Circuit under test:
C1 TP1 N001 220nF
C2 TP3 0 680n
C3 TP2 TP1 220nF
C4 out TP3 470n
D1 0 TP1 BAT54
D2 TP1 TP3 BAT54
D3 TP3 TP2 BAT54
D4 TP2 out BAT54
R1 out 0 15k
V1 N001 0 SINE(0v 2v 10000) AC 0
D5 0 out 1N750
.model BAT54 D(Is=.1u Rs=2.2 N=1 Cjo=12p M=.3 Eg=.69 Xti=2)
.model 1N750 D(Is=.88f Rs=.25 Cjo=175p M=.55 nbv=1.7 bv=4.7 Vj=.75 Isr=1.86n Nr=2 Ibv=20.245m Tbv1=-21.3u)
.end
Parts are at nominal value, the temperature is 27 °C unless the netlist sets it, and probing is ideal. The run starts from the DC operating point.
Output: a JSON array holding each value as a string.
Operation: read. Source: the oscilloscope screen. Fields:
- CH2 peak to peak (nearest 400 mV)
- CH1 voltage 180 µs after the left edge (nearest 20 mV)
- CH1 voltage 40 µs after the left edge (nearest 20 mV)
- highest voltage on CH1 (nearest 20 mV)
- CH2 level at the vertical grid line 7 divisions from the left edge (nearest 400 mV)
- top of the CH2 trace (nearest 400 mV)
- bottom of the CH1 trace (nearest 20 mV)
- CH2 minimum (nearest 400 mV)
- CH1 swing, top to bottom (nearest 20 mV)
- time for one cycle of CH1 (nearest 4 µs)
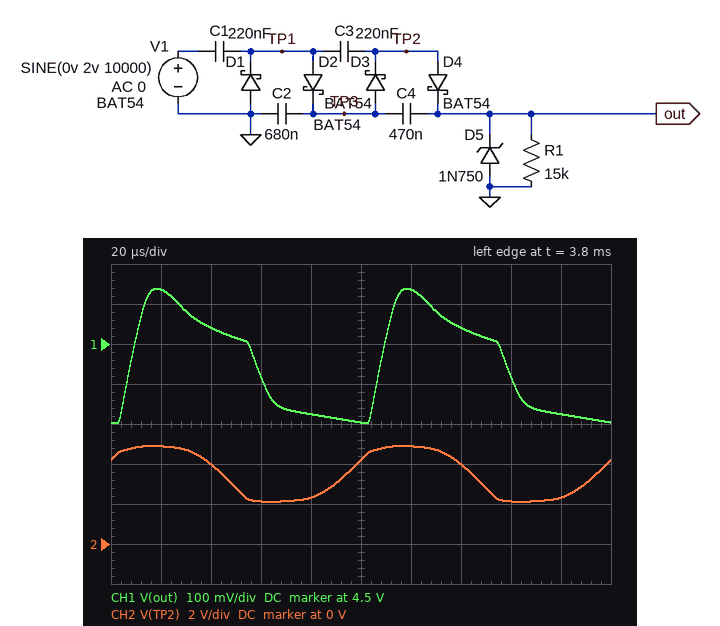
["2.8 V", "4.32 V", "4.54 V", "4.64 V", "4.0 V", "4.8 V", "4.30 V", "2.0 V", "340 mV", "100 µs"]
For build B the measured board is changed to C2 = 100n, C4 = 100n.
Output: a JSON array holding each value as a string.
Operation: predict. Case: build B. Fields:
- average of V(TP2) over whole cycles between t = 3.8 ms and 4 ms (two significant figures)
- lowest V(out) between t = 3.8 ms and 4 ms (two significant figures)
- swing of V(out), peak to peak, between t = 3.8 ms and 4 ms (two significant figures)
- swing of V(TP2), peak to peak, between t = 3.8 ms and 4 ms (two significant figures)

["3.3 V", "3.4 V", "1.2 V", "3.2 V"]
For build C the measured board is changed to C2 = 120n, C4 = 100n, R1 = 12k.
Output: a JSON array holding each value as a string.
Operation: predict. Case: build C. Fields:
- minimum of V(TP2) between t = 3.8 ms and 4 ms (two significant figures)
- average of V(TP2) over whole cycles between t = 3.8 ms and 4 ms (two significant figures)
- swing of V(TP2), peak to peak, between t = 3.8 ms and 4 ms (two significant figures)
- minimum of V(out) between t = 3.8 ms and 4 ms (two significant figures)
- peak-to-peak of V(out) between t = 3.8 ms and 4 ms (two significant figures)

["1.8 V", "3.3 V", "3.1 V", "3.4 V", "1.2 V"]
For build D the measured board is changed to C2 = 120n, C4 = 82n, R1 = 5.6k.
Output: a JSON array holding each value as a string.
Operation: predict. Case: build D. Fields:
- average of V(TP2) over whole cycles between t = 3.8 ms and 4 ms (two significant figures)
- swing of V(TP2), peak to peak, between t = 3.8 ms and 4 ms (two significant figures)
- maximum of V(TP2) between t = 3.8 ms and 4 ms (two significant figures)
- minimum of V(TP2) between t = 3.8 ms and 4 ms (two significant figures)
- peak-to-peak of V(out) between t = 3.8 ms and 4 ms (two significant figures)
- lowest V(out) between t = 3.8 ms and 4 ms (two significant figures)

["3.2 V", "3.1 V", "4.8 V", "1.7 V", "1.6 V", "3.0 V"]
